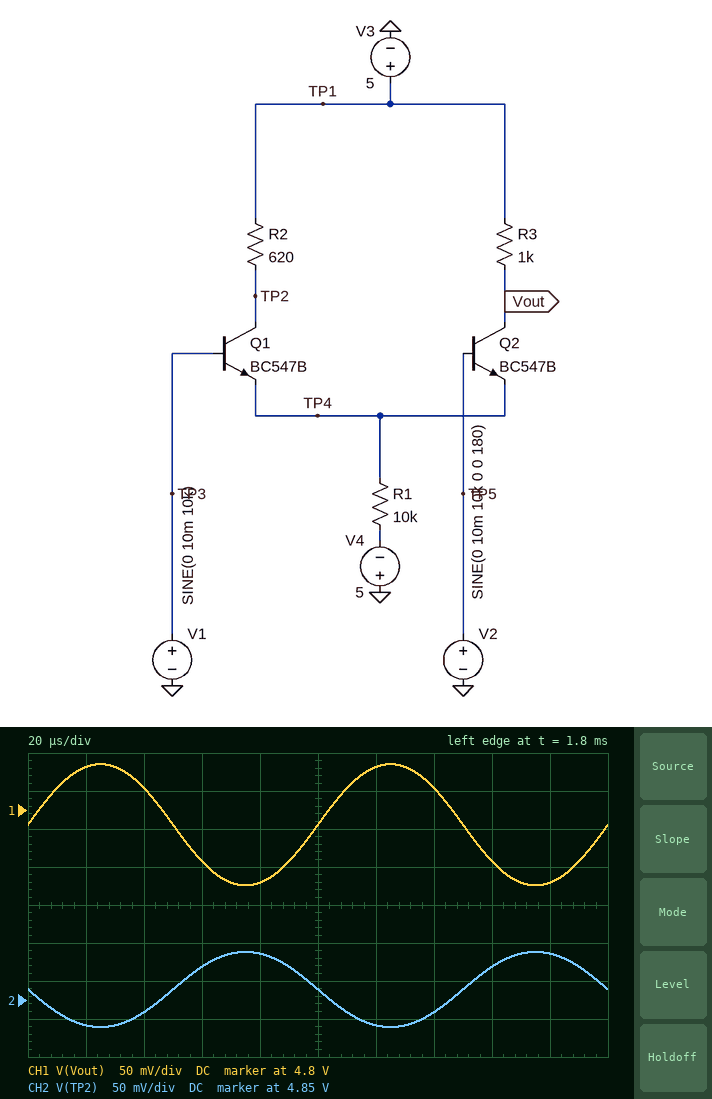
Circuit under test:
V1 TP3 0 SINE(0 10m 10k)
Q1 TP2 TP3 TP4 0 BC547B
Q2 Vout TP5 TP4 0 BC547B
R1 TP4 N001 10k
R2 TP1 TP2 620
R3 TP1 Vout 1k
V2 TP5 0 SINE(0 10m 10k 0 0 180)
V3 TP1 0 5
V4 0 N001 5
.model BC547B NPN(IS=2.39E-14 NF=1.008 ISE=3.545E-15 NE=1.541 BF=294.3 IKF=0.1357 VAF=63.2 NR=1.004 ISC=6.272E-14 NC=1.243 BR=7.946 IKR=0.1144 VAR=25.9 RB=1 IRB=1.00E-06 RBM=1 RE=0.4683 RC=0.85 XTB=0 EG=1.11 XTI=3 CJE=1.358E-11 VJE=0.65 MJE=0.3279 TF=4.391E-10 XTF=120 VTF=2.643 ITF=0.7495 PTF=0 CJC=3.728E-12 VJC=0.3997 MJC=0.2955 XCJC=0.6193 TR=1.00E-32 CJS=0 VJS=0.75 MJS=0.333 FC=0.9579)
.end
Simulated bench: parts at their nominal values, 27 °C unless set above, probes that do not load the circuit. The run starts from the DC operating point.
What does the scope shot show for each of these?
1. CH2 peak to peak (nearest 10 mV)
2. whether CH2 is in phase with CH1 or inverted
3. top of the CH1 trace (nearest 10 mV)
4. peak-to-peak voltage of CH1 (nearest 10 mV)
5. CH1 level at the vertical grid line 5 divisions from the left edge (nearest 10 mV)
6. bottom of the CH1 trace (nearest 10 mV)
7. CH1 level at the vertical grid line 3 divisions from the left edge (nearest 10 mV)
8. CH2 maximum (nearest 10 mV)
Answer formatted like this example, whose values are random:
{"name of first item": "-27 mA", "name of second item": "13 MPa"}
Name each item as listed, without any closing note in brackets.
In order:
{"CH2 peak to peak": "100 mV", "whether CH2 is in phase with CH1 or inverted": "inverted", "top of the CH1 trace": "4.86 V", "peak-to-peak voltage of CH1": "160 mV", "CH1 level at the vertical grid line 5 divisions from the left edge": "4.78 V", "bottom of the CH1 trace": "4.70 V", "CH1 level at the vertical grid line 3 divisions from the left edge": "4.73 V", "CH2 maximum": "4.91 V"}
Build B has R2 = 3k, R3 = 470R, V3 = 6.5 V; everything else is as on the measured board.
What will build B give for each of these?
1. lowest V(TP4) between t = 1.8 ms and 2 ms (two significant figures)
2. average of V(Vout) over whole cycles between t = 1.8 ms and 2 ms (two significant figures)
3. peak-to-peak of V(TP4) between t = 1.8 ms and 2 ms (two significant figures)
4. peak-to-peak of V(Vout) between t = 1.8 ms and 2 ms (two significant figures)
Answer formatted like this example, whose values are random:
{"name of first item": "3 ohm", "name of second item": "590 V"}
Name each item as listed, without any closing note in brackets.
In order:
{"lowest V(TP4) between t = 1.8 ms and 2 ms": "-600 mV", "average of V(Vout) over whole cycles between t = 1.8 ms and 2 ms": "6.4 V", "peak-to-peak of V(TP4) between t = 1.8 ms and 2 ms": "1.9 mV", "peak-to-peak of V(Vout) between t = 1.8 ms and 2 ms": "75 mV"}
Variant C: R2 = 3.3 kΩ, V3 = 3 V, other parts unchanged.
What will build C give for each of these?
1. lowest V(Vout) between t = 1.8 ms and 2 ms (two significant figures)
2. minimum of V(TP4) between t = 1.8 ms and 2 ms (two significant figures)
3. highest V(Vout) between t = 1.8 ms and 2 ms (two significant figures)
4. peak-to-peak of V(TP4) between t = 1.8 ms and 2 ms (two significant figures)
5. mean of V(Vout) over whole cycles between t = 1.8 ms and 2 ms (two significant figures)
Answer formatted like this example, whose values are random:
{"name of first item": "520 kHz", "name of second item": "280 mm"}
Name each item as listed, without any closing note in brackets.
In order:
{"lowest V(Vout) between t = 1.8 ms and 2 ms": "2.7 V", "minimum of V(TP4) between t = 1.8 ms and 2 ms": "-600 mV", "highest V(Vout) between t = 1.8 ms and 2 ms": "2.9 V", "peak-to-peak of V(TP4) between t = 1.8 ms and 2 ms": "1.9 mV", "mean of V(Vout) over whole cycles between t = 1.8 ms and 2 ms": "2.8 V"}
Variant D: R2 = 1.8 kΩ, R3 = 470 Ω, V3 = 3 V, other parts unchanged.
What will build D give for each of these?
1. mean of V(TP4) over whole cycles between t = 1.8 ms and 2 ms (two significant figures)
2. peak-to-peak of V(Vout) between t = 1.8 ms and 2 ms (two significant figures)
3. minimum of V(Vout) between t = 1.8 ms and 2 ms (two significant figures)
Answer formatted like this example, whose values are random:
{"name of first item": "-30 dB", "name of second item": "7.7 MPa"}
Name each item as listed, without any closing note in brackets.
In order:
{"mean of V(TP4) over whole cycles between t = 1.8 ms and 2 ms": "-600 mV", "peak-to-peak of V(Vout) between t = 1.8 ms and 2 ms": "75 mV", "minimum of V(Vout) between t = 1.8 ms and 2 ms": "2.9 V"}
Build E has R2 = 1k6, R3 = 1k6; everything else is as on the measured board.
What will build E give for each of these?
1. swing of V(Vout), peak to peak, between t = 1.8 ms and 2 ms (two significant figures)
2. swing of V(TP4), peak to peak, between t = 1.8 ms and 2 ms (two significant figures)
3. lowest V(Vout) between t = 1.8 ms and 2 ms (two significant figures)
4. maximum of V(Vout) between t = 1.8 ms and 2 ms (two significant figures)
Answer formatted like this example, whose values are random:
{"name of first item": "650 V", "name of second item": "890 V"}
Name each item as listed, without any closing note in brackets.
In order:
{"swing of V(Vout), peak to peak, between t = 1.8 ms and 2 ms": "250 mV", "swing of V(TP4), peak to peak, between t = 1.8 ms and 2 ms": "1.8 mV", "lowest V(Vout) between t = 1.8 ms and 2 ms": "4.5 V", "maximum of V(Vout) between t = 1.8 ms and 2 ms": "4.8 V"}
